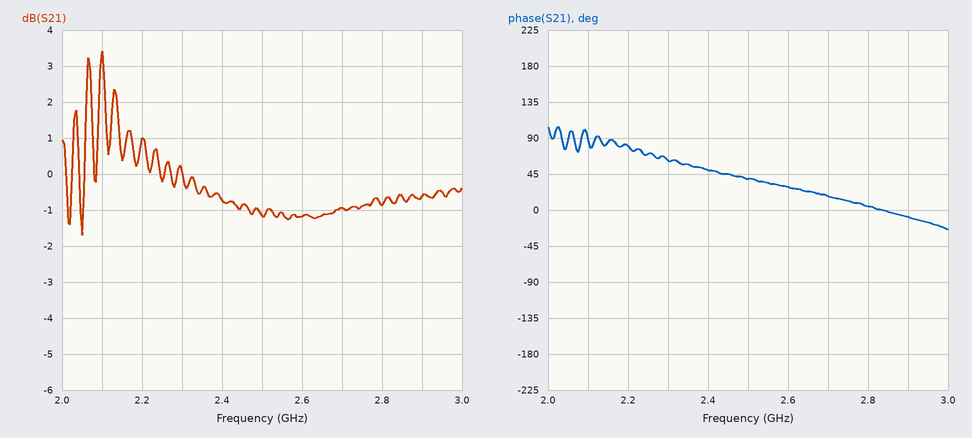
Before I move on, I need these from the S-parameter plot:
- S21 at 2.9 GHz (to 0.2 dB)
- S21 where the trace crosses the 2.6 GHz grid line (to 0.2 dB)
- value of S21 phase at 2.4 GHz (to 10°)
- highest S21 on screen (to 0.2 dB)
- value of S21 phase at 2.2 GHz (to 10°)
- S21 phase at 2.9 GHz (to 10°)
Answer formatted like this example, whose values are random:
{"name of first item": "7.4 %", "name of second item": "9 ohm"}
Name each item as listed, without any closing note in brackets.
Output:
{"S21 at 2.9 GHz": "-0.6 dB", "S21 where the trace crosses the 2.6 GHz grid line": "-1.2 dB", "value of S21 phase at 2.4 GHz": "50°", "highest S21 on screen": "3.4 dB", "value of S21 phase at 2.2 GHz": "80°", "S21 phase at 2.9 GHz": "-10°"}
